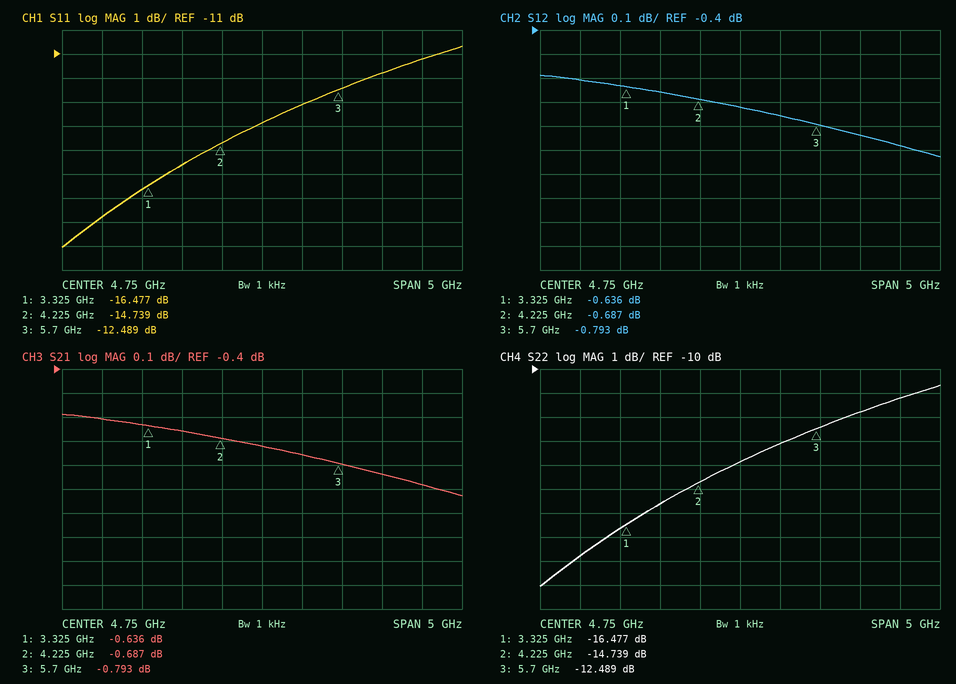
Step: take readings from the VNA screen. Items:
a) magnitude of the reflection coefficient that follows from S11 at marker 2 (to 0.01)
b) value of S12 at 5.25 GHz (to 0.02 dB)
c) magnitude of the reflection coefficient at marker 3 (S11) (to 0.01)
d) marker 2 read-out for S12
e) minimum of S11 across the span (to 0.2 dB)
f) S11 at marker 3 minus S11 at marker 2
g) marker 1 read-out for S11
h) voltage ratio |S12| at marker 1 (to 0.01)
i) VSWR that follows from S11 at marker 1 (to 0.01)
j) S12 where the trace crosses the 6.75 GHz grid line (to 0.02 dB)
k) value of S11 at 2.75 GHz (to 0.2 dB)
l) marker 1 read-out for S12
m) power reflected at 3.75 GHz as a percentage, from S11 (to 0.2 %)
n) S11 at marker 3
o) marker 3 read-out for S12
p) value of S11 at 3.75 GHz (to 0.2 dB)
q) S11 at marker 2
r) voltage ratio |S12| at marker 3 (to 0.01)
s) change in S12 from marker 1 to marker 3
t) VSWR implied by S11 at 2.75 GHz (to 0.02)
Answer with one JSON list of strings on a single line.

["0.18", "-0.76 dB", "0.24", "-0.687 dB", "-19.0 dB", "2.250 dB", "-16.477 dB", "0.93", "1.35", "-0.88 dB", "-17.8 dB", "-0.636 dB", "2.8 %", "-12.489 dB", "-0.793 dB", "-15.6 dB", "-14.739 dB", "0.91", "-0.157 dB", "1.30"]
